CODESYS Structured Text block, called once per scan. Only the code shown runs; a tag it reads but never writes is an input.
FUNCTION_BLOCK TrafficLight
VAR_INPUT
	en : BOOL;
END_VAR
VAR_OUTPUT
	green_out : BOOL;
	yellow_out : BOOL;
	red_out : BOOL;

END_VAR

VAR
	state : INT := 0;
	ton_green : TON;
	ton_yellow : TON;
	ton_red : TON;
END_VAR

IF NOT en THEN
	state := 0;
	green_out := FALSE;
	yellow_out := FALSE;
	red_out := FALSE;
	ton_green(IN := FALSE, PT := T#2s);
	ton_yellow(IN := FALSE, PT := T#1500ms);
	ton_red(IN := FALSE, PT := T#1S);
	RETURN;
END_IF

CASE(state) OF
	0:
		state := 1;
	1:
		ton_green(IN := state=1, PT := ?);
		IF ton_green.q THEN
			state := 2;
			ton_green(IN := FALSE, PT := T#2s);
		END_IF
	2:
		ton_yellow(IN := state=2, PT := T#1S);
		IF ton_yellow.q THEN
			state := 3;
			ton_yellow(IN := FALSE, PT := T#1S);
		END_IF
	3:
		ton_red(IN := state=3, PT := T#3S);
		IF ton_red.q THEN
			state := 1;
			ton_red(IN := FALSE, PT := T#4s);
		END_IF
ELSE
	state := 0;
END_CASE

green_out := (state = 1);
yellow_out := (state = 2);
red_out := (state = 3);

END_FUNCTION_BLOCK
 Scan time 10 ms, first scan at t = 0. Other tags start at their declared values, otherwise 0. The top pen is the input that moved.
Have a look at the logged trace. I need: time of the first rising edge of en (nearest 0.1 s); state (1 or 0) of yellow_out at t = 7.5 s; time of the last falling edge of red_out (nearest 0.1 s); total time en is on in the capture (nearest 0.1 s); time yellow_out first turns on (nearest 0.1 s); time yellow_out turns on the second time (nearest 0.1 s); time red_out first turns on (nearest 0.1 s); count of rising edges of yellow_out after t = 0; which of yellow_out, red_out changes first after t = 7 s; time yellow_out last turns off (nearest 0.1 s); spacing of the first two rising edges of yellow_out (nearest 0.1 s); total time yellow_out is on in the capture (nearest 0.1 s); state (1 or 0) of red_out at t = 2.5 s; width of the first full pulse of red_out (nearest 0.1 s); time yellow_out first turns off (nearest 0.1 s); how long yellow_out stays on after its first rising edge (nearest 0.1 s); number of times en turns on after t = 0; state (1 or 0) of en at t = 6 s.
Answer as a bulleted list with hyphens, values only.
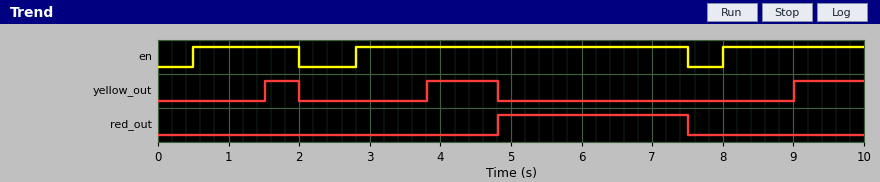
- 0.5 s
- 0
- 7.5 s
- 8.2 s
- 1.5 s
- 3.8 s
- 4.8 s
- 3
- red_out
- 4.8 s
- 2.3 s
- 2.5 s
- 0
- 2.7 s
- 2.0 s
- 0.5 s
- 3
- 1
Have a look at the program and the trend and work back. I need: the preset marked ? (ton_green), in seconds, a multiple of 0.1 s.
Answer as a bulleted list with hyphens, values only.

- 1.0 s
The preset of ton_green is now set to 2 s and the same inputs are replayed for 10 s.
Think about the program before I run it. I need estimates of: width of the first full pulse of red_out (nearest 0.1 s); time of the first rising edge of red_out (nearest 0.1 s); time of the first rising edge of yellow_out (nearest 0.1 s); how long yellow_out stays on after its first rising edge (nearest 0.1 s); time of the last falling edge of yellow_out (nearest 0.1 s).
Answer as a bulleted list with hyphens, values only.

- 1.7 s
- 5.8 s
- 4.8 s
- 1.0 s
- 5.8 s
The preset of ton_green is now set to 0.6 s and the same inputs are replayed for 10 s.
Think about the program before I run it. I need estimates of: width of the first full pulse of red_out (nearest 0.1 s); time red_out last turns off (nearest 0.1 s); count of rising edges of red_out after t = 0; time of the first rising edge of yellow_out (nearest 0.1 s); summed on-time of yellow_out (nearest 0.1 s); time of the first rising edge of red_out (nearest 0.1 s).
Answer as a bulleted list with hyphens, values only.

- 3.0 s
- 7.4 s
- 2
- 1.1 s
- 2.9 s
- 4.4 s
